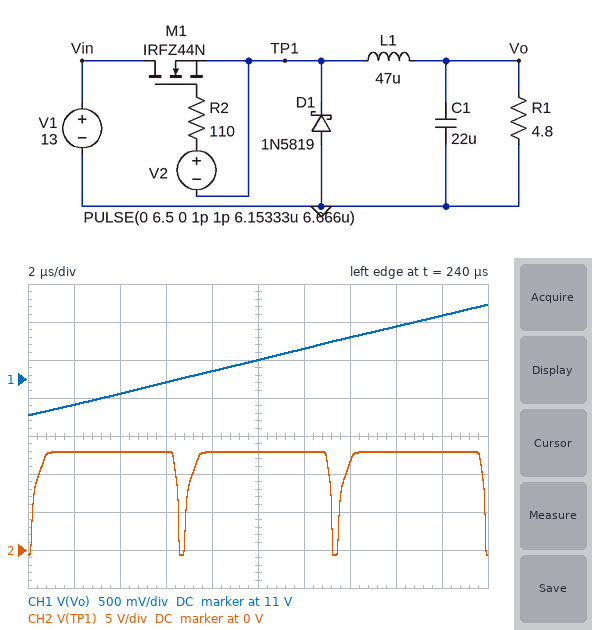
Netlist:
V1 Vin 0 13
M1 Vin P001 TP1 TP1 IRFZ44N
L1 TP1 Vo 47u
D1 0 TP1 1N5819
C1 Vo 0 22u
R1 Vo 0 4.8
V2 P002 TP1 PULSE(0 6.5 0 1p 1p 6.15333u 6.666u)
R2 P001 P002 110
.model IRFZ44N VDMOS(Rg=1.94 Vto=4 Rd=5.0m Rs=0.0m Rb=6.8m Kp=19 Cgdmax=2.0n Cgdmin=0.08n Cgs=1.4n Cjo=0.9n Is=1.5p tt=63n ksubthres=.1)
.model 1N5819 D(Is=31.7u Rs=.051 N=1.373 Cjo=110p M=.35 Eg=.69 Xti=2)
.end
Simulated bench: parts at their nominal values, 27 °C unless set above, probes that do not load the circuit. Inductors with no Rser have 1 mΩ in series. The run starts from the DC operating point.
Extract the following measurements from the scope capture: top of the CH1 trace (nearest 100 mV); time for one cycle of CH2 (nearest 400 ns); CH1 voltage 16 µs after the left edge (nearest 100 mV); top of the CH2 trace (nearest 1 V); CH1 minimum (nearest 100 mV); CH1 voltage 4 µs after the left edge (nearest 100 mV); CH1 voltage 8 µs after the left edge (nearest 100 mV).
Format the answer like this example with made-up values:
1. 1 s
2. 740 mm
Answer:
1. 12.0 V
2. 6.8 µs
3. 11.7 V
4. 13 V
5. 10.5 V
6. 10.8 V
7. 11.1 V
